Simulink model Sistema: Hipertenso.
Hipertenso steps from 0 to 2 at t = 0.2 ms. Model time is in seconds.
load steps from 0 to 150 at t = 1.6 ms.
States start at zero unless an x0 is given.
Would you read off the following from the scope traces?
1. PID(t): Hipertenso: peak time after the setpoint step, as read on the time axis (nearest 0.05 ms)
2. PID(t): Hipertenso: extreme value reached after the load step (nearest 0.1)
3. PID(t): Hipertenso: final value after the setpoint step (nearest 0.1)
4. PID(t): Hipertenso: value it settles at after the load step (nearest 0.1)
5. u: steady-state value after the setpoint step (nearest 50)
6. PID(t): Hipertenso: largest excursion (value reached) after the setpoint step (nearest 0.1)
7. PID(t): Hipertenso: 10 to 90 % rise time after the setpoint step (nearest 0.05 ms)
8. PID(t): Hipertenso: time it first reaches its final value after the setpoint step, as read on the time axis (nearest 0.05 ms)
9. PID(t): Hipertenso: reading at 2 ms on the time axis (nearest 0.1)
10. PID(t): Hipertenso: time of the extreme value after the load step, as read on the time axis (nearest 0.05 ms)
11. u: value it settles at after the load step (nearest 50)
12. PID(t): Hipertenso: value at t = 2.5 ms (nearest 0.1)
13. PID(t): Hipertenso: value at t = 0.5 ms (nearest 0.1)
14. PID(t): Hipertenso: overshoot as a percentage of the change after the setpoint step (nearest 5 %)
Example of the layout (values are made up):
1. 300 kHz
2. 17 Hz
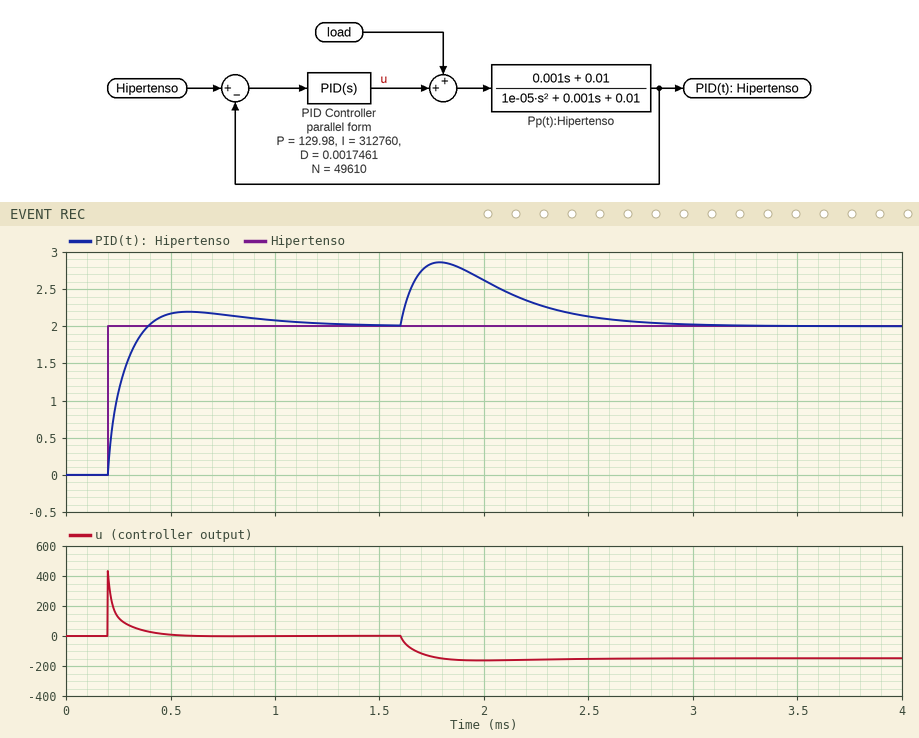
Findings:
1. 0.60 ms
2. 2.9
3. 2.0
4. 2.0
5. 0
6. 2.2
7. 0.15 ms
8. 0.40 ms
9. 2.6
10. 1.80 ms
11. -150
12. 2.1
13. 2.2
14. 10 %
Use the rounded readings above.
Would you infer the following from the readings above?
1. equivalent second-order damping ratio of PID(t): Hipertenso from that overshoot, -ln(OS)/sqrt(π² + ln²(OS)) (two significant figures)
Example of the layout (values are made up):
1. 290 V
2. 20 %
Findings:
1. 0.59
